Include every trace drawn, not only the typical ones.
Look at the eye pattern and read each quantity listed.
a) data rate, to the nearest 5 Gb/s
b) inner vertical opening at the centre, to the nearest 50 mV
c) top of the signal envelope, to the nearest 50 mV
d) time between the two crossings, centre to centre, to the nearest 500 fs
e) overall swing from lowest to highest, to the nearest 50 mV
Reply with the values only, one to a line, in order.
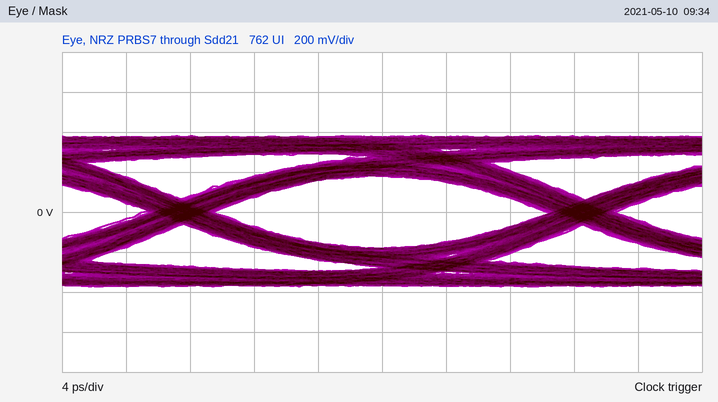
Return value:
40 Gb/s
350 mV
400 mV
25.0 ps
750 mV
